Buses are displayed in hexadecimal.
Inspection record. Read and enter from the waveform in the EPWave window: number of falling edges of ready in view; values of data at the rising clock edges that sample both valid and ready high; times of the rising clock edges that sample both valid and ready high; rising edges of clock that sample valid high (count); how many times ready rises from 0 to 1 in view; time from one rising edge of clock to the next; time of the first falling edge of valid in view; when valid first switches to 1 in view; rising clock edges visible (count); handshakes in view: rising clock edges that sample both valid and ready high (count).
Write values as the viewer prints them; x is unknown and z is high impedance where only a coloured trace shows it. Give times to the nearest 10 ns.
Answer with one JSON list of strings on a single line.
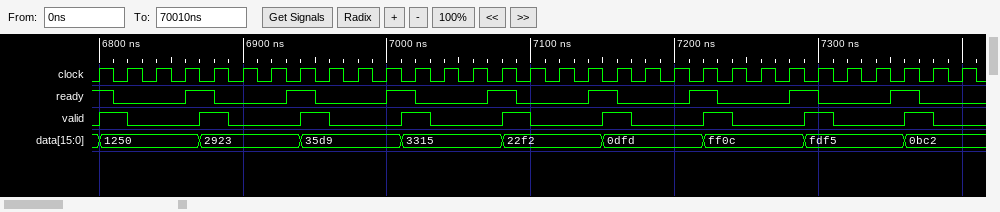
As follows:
["9", "2923, 3315, 0dfd, fdf5", "6880 ns, 7020 ns, 7160 ns, 7300 ns", "9", "8", "20 ns", "6820 ns", "6800 ns", "31", "4"]
